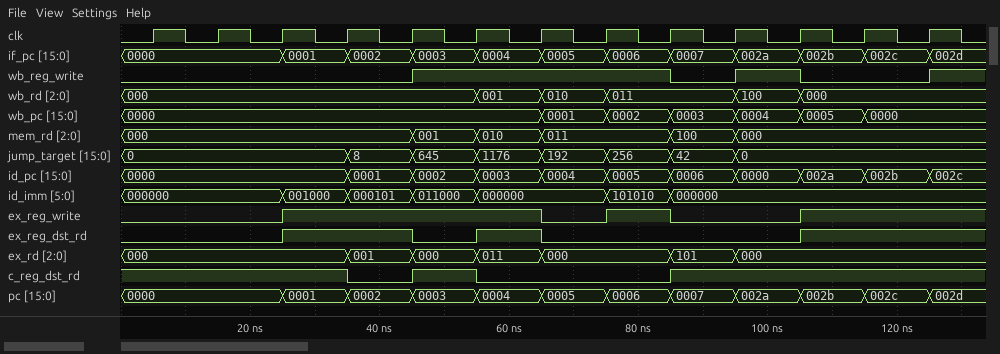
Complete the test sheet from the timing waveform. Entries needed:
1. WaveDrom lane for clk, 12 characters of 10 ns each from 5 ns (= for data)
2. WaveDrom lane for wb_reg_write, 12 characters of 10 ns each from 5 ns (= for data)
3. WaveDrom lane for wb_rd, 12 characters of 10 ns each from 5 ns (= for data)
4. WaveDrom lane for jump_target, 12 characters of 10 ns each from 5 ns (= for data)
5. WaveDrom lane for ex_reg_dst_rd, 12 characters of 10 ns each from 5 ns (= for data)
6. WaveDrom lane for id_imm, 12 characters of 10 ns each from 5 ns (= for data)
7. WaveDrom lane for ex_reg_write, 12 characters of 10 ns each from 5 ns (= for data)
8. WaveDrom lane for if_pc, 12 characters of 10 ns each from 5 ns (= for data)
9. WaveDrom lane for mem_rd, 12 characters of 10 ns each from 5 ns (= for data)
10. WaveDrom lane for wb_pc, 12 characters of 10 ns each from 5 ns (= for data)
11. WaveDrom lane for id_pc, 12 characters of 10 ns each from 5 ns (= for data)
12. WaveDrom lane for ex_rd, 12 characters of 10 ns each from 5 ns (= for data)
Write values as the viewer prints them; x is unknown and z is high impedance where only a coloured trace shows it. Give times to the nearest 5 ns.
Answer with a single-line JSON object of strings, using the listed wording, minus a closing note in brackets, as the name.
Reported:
{"WaveDrom lane for clk, 12 characters of 10 ns each from 5 ns": "{name: 'clk', wave: 'p...........'}", "WaveDrom lane for wb_reg_write, 12 characters of 10 ns each from 5 ns": "{name: 'wb_reg_write', wave: '0...1...010.'}", "WaveDrom lane for wb_rd, 12 characters of 10 ns each from 5 ns": "{name: 'wb_rd', wave: '=....===.==.', data: '000 001 010 011 100 000'}", "WaveDrom lane for jump_target, 12 characters of 10 ns each from 5 ns": "{name: 'jump_target', wave: '=..=======..', data: '0 8 645 1176 192 256 42 0'}", "WaveDrom lane for ex_reg_dst_rd, 12 characters of 10 ns each from 5 ns": "{name: 'ex_reg_dst_rd', wave: '0.1.010...1.'}", "WaveDrom lane for id_imm, 12 characters of 10 ns each from 5 ns": "{name: 'id_imm', wave: '=.====.==...', data: '000000 001000 000101 011000 000000 101010 000000'}", "WaveDrom lane for ex_reg_write, 12 characters of 10 ns each from 5 ns": "{name: 'ex_reg_write', wave: '0.1...010.1.'}", "WaveDrom lane for if_pc, 12 characters of 10 ns each from 5 ns": "{name: 'if_pc', wave: '=.==========', data: '0000 0001 0002 0003 0004 0005 0006 0007 002a 002b 002c'}", "WaveDrom lane for mem_rd, 12 characters of 10 ns each from 5 ns": "{name: 'mem_rd', wave: '=...===.==..', data: '000 001 010 011 100 000'}", "WaveDrom lane for wb_pc, 12 characters of 10 ns each from 5 ns": "{name: 'wb_pc', wave: '=.....======', data: '0000 0001 0002 0003 0004 0005 0000'}", "WaveDrom lane for id_pc, 12 characters of 10 ns each from 5 ns": "{name: 'id_pc', wave: '=..=========', data: '0000 0001 0002 0003 0004 0005 0006 0000 002a 002b'}", "WaveDrom lane for ex_rd, 12 characters of 10 ns each from 5 ns": "{name: 'ex_rd', wave: '=..====.==..', data: '000 001 000 011 000 101 000'}"}
